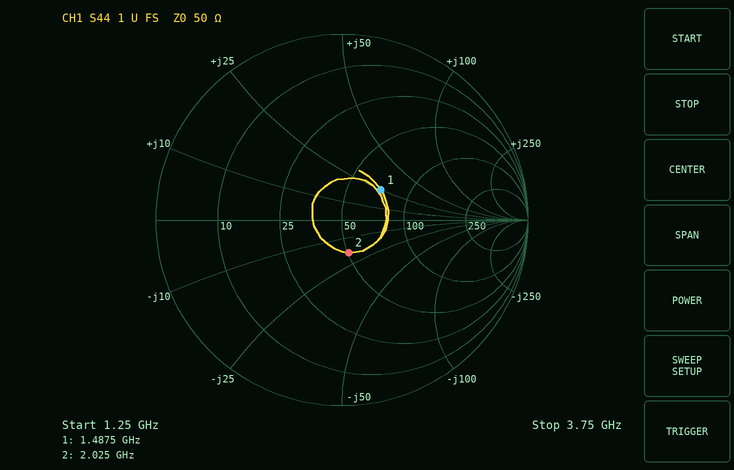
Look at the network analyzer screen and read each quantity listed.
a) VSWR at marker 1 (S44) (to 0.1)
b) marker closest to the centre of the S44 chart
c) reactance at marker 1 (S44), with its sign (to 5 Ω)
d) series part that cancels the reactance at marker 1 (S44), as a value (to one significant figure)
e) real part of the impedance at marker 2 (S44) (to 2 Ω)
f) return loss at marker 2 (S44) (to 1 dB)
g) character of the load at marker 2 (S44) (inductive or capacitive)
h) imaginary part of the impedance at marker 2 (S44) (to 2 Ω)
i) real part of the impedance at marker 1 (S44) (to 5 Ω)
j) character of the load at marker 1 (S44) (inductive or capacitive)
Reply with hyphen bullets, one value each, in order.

- 1.7
- marker 2
- +25 Ω
- 4 pF
- 50 Ω
- 15 dB
- capacitive
- -18 Ω
- 70 Ω
- inductive
